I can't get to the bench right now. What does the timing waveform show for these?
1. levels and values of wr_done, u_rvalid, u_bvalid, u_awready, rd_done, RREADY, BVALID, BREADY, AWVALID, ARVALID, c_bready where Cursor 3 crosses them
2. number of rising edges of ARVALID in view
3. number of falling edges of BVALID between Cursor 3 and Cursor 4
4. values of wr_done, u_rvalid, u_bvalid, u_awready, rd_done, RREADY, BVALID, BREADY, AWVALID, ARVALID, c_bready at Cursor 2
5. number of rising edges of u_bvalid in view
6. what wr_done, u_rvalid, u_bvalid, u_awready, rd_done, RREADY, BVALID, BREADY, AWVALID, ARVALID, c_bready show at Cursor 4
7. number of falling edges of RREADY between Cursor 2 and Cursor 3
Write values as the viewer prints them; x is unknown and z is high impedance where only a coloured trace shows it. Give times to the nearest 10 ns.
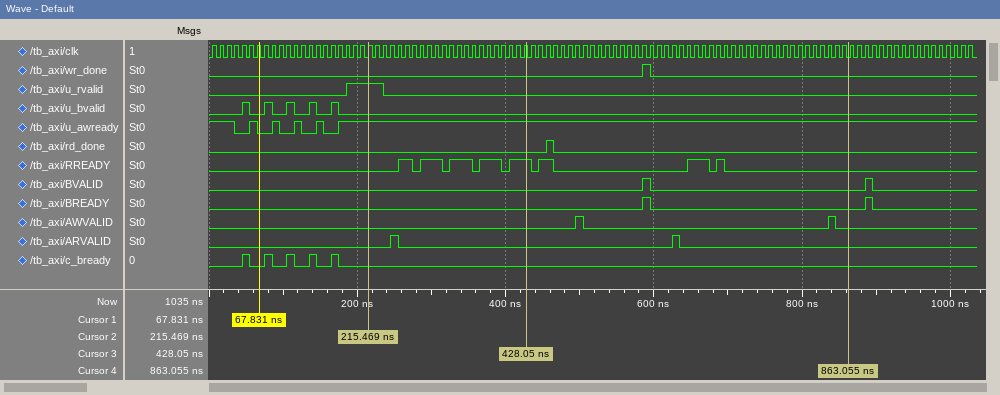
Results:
wr_done=0, u_rvalid=0, u_bvalid=0, u_awready=1, rd_done=0, RREADY=1, BVALID=0, BREADY=0, AWVALID=0, ARVALID=0, c_bready=0
2
1
wr_done=0, u_rvalid=1, u_bvalid=0, u_awready=1, rd_done=0, RREADY=0, BVALID=0, BREADY=0, AWVALID=0, ARVALID=0, c_bready=0
5
wr_done=0, u_rvalid=0, u_bvalid=0, u_awready=1, rd_done=0, RREADY=0, BVALID=0, BREADY=0, AWVALID=0, ARVALID=0, c_bready=0
4
